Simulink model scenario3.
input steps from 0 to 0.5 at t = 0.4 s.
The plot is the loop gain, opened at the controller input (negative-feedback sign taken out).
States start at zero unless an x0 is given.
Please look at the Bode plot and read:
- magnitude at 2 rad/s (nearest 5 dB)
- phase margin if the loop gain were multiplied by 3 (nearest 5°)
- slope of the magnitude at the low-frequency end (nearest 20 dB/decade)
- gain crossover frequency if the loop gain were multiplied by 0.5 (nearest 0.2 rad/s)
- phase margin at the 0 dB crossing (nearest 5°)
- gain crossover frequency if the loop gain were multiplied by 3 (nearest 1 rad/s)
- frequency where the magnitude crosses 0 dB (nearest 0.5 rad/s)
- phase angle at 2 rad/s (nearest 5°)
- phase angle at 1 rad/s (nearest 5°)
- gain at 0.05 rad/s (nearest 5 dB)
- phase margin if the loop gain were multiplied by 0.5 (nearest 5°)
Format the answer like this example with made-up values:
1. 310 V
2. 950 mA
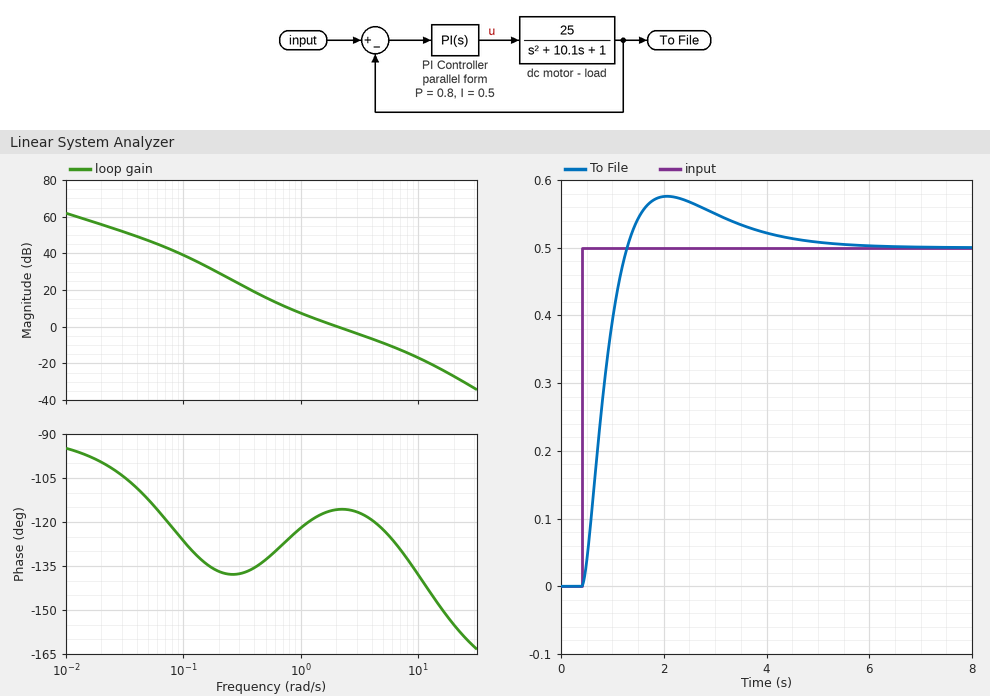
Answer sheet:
1. 0 dB
2. 55°
3. -20 dB/decade
4. 1.2 rad/s
5. 65°
6. 5 rad/s
7. 2.0 rad/s
8. -115°
9. -120°
10. 45 dB
11. 60°
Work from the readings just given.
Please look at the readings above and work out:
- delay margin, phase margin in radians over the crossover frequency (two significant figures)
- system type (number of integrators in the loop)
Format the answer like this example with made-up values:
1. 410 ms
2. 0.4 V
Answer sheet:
1. 0.57 s
2. 1
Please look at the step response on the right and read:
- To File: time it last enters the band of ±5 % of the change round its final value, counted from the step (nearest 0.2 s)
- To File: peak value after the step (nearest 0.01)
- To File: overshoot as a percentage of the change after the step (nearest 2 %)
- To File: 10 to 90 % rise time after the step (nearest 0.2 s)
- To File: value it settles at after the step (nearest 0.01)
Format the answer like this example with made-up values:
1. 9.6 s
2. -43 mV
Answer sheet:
1. 3.4 s
2. 0.58
3. 16 %
4. 0.6 s
5. 0.50
